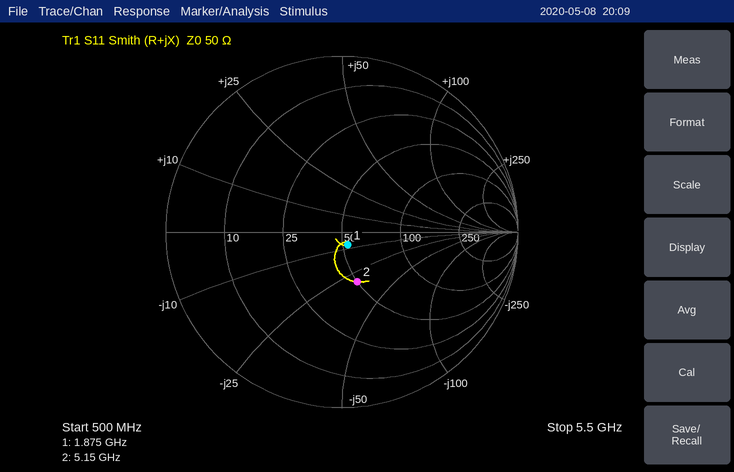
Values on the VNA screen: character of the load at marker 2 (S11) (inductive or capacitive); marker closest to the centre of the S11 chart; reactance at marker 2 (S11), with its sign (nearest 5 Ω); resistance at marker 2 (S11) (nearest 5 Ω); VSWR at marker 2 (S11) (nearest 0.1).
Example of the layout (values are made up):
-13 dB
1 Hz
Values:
capacitive
marker 1
-30 Ω
50 Ω
1.8
